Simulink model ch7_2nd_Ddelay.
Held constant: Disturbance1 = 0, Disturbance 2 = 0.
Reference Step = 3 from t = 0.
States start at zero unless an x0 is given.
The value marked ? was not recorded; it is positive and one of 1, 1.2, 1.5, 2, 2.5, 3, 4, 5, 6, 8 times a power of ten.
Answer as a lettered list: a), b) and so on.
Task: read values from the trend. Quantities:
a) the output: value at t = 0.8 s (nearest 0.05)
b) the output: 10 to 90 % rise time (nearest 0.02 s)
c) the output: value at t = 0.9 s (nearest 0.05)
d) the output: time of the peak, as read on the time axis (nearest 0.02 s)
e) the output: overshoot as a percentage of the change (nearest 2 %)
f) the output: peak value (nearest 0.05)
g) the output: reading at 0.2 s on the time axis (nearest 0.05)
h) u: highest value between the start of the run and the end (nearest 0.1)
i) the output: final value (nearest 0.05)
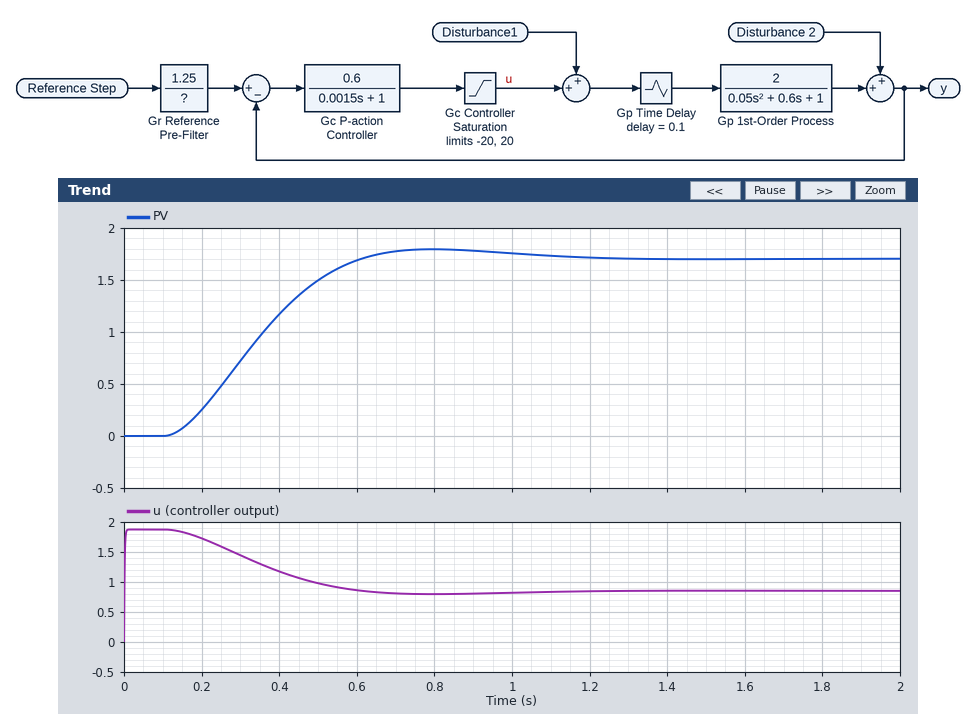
a) 1.80
b) 0.34 s
c) 1.80
d) 0.80 s
e) 6 %
f) 1.80
g) 0.25
h) 1.9
i) 1.70
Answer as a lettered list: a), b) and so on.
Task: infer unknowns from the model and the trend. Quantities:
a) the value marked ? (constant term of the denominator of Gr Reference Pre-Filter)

a) 1.2
